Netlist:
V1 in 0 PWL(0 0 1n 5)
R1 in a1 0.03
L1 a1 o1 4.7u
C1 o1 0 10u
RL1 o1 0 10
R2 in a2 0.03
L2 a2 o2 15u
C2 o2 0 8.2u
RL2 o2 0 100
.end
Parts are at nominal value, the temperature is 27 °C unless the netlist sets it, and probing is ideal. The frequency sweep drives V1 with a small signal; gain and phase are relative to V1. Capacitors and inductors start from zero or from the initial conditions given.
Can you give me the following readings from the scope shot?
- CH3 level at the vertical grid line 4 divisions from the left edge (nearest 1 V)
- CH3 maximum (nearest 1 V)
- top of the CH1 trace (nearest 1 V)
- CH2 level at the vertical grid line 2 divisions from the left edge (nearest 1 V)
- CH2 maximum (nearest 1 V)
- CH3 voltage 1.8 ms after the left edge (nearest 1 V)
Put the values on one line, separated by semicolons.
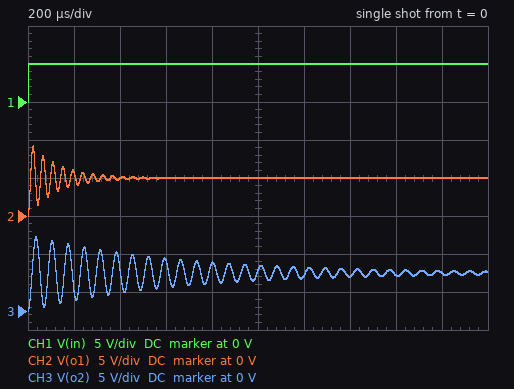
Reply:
6 V; 10 V; 5 V; 5 V; 9 V; 5 V
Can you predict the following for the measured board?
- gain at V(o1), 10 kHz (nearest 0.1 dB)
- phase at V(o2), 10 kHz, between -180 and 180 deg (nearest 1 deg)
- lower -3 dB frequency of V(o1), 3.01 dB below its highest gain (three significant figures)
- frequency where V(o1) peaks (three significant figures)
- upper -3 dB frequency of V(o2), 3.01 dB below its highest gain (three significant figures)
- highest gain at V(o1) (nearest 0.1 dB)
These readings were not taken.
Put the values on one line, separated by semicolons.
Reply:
1.7 dB; -3 deg; 21.8 kHz; 23.2 kHz; 14.6 kHz; 19.0 dB
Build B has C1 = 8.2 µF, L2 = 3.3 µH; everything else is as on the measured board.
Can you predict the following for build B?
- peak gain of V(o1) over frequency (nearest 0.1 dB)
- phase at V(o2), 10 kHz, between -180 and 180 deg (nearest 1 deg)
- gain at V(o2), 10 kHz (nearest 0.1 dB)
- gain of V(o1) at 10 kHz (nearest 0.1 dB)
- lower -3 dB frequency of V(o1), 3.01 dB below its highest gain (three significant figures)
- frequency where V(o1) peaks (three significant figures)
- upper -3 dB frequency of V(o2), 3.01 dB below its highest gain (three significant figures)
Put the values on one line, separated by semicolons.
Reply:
18.8 dB; -1 deg; 1.0 dB; 1.4 dB; 24.1 kHz; 25.6 kHz; 31.4 kHz
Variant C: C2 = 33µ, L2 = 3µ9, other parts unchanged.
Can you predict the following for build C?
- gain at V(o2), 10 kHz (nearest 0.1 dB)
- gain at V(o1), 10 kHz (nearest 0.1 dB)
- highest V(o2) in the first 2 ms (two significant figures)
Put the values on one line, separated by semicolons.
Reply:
6.1 dB; 1.7 dB; 9.3 V
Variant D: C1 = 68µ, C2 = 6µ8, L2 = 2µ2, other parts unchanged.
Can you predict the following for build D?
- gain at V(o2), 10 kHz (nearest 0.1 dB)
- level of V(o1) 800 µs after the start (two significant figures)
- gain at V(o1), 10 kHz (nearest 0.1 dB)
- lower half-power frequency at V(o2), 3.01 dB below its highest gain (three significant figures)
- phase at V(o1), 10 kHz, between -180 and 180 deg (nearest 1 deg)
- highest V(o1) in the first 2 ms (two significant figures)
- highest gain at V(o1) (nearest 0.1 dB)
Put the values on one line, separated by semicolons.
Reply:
0.5 dB; 4.8 V; 10.4 dB; 39.9 kHz; -149 deg; 9.0 V; 17.1 dB
